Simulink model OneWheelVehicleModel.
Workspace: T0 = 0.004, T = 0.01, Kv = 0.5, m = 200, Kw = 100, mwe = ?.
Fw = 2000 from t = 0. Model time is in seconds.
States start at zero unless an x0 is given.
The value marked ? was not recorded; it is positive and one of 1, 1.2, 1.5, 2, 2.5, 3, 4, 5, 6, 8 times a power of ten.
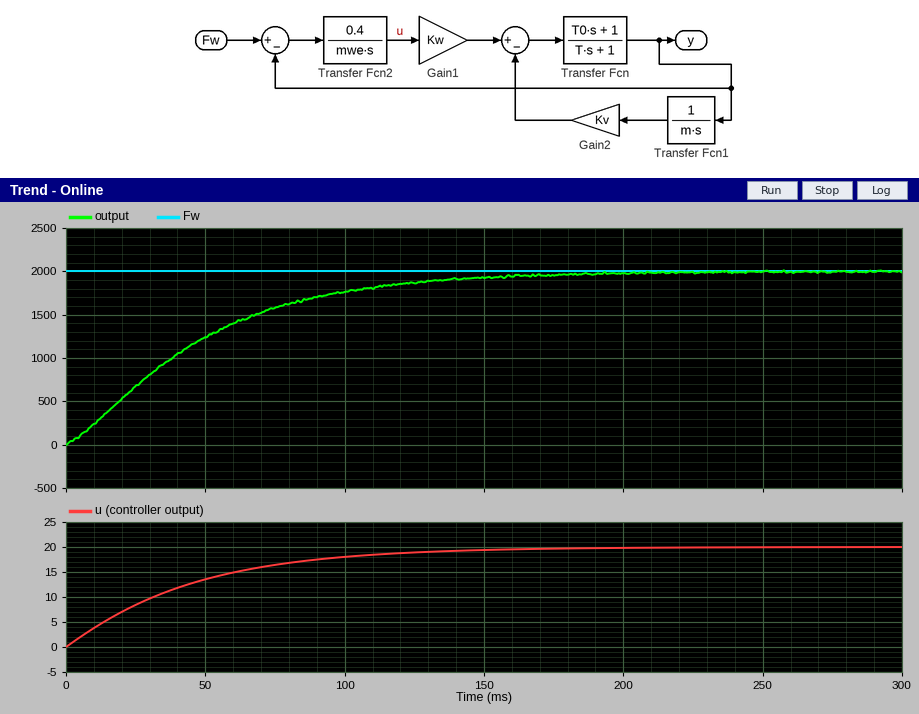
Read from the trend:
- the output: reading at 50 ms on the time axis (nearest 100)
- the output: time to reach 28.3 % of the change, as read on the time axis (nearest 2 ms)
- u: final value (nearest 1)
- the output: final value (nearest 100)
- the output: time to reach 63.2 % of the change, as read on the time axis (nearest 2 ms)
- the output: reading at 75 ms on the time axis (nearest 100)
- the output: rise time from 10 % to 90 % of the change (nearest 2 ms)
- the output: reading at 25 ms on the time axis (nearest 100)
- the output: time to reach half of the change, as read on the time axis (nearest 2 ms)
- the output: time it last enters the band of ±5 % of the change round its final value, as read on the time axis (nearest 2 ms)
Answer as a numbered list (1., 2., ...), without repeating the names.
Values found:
1. 1200
2. 22 ms
3. 20
4. 2000
5. 52 ms
6. 1600
7. 98 ms
8. 700
9. 38 ms
10. 136 ms
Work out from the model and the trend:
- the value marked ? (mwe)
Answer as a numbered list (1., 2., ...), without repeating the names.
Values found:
1. 2
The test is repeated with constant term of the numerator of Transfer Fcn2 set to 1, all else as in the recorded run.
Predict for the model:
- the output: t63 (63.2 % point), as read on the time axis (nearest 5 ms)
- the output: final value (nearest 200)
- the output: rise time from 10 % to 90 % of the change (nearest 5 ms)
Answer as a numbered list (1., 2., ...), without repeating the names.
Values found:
1. 25 ms
2. 2000
3. 35 ms
